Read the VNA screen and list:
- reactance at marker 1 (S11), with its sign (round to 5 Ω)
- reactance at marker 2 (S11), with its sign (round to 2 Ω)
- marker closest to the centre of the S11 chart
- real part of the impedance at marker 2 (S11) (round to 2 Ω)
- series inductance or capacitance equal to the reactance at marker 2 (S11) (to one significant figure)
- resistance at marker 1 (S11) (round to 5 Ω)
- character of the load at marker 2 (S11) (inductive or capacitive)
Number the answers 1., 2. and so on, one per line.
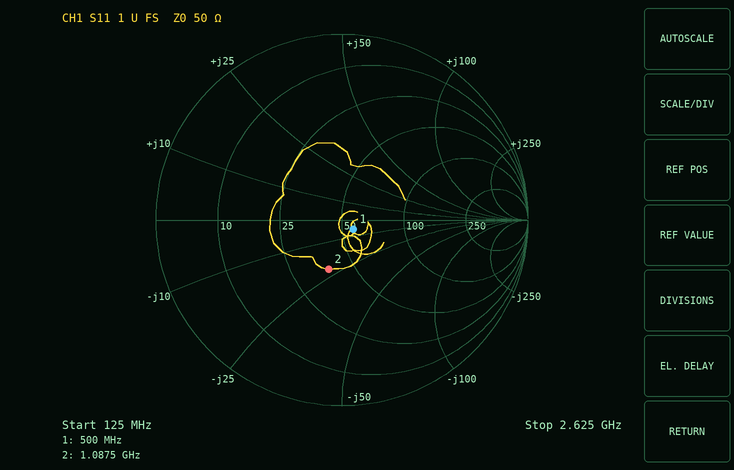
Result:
1. -5 Ω
2. -22 Ω
3. marker 1
4. 38 Ω
5. 7 pF
6. 55 Ω
7. capacitive
